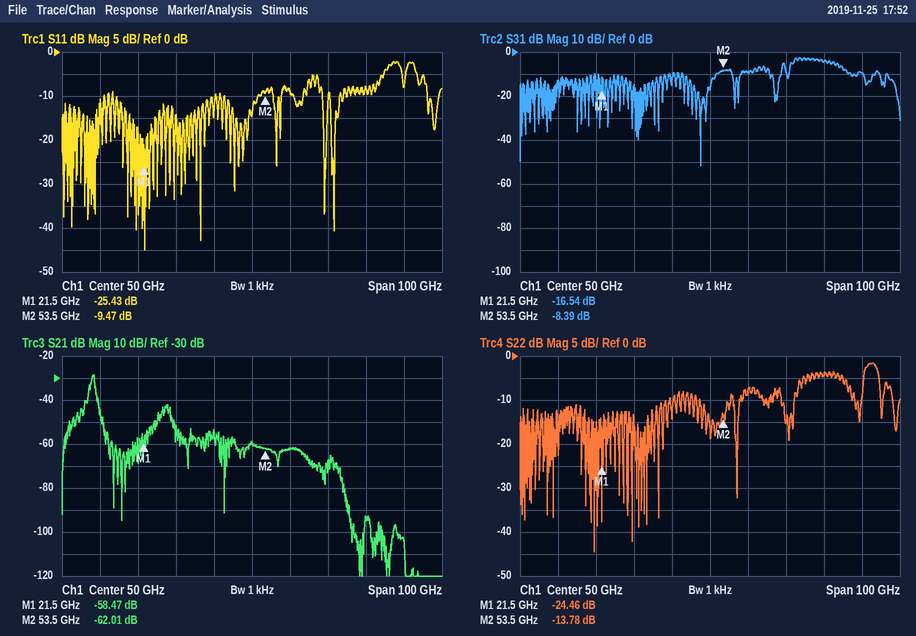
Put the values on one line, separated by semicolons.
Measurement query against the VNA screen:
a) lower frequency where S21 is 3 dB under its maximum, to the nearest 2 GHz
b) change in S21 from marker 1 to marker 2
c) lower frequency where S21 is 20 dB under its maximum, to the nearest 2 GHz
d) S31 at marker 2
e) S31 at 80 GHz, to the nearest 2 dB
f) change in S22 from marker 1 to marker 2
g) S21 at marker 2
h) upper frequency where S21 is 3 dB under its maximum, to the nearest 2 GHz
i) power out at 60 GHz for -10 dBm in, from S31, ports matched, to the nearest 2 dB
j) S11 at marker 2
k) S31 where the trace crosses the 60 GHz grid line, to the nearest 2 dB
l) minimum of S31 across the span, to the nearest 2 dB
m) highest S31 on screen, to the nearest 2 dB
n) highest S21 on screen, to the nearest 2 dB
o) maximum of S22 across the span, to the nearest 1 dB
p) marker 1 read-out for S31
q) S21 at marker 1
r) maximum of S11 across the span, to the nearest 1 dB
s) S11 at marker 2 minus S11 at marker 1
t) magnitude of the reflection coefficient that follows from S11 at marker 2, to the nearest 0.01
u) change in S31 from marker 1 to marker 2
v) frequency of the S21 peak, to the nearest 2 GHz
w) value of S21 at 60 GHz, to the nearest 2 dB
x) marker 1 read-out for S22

8 GHz; -3.54 dB; 4 GHz; -8.39 dB; -4 dB; 10.68 dB; -62.01 dB; 8 GHz; -20 dBm; -9.47 dB; -10 dB; -52 dB; -2 dB; -28 dB; -2 dB; -16.54 dB; -58.47 dB; -2 dB; 15.96 dB; 0.34; 8.15 dB; 8 GHz; -62 dB; -24.46 dB
